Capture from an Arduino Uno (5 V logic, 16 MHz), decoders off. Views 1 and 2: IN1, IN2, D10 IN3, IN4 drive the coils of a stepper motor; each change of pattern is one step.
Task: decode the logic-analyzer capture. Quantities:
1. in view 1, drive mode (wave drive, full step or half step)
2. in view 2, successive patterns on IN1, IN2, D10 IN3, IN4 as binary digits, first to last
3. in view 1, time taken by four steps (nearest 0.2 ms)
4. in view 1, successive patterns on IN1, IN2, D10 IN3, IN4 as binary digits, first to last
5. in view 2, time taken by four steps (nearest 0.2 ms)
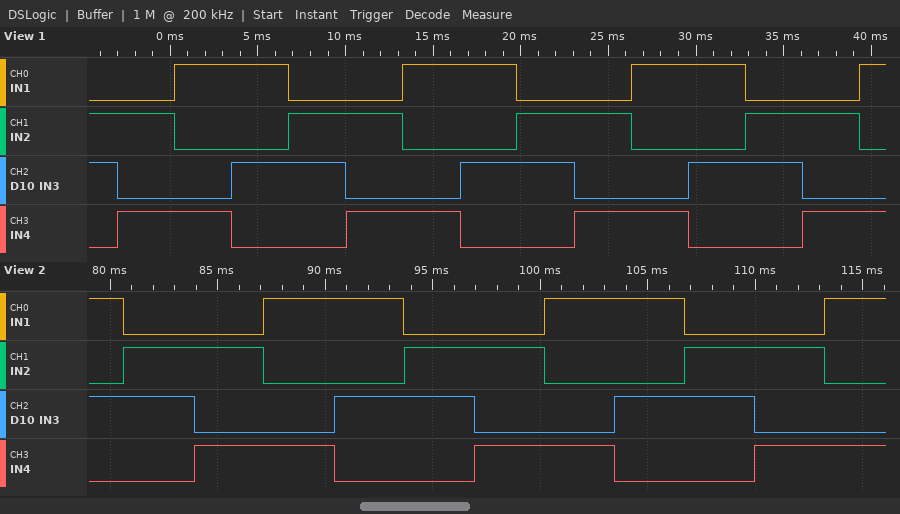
full step
1010 0110 0101 1001 1010 0110 0101 1001 1010 0110 0101 1001
13.0 ms
0110 0101 1001 1010 0110 0101 1001 1010 0110 0101 1001 1010 0110 0101 1001
13.0 ms
